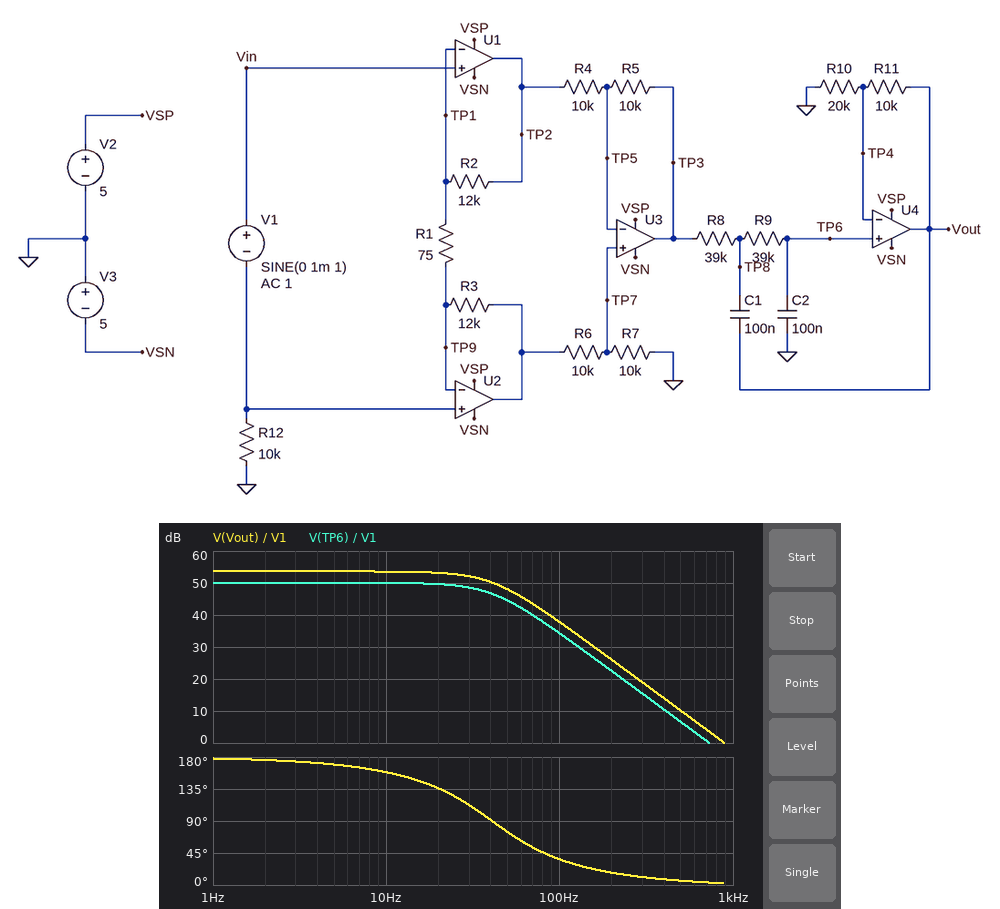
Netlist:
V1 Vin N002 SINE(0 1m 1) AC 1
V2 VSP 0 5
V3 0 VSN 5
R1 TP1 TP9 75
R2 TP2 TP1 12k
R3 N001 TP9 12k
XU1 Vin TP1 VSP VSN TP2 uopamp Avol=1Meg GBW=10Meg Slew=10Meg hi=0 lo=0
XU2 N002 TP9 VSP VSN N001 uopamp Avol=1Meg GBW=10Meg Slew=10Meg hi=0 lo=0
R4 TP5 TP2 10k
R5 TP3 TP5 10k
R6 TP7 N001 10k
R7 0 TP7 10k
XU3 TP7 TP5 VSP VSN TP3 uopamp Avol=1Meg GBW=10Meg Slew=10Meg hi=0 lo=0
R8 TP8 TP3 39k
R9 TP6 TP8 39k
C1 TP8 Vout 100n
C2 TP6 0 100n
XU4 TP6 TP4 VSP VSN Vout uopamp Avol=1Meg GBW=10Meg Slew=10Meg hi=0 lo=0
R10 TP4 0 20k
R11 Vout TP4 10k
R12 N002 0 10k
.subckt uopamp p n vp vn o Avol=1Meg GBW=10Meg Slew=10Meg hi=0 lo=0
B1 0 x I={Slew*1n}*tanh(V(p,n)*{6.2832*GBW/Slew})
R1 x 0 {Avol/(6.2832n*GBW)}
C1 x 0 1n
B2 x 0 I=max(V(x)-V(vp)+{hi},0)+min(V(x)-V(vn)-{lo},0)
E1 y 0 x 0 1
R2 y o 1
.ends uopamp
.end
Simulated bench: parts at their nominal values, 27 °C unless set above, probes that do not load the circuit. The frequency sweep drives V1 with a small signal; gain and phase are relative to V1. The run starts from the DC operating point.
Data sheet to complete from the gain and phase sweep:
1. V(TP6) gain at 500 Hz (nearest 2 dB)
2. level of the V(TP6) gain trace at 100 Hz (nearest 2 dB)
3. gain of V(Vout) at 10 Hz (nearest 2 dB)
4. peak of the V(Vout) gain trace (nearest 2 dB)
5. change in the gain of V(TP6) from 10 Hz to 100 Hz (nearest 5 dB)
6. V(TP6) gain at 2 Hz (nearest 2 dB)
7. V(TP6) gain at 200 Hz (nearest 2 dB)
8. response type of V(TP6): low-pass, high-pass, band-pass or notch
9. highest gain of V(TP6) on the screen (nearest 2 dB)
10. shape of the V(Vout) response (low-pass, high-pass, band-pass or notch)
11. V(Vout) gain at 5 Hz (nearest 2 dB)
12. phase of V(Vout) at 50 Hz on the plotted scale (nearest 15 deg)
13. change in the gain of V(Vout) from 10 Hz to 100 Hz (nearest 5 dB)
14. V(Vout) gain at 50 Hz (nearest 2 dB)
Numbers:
6 dB
34 dB
54 dB
54 dB
-15 dB
50 dB
22 dB
low-pass
50 dB
low-pass
54 dB
75 deg
-15 dB
48 dB
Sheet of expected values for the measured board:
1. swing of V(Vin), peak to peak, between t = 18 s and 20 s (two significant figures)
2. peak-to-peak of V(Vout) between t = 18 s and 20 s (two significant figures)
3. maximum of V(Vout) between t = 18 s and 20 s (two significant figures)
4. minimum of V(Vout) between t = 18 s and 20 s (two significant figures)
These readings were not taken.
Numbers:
2.0 mV
960 mV
480 mV
-480 mV
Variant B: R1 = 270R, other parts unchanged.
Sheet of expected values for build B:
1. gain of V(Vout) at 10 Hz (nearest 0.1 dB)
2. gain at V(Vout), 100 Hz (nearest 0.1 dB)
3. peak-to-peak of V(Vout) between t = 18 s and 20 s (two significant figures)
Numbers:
42.5 dB
26.7 dB
270 mV
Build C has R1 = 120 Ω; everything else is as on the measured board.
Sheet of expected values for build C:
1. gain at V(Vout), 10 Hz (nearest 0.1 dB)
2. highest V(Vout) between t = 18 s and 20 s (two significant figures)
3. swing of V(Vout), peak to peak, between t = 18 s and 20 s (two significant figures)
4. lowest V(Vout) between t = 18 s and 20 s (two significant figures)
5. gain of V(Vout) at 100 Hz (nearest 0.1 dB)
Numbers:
49.5 dB
300 mV
600 mV
-300 mV
33.7 dB
